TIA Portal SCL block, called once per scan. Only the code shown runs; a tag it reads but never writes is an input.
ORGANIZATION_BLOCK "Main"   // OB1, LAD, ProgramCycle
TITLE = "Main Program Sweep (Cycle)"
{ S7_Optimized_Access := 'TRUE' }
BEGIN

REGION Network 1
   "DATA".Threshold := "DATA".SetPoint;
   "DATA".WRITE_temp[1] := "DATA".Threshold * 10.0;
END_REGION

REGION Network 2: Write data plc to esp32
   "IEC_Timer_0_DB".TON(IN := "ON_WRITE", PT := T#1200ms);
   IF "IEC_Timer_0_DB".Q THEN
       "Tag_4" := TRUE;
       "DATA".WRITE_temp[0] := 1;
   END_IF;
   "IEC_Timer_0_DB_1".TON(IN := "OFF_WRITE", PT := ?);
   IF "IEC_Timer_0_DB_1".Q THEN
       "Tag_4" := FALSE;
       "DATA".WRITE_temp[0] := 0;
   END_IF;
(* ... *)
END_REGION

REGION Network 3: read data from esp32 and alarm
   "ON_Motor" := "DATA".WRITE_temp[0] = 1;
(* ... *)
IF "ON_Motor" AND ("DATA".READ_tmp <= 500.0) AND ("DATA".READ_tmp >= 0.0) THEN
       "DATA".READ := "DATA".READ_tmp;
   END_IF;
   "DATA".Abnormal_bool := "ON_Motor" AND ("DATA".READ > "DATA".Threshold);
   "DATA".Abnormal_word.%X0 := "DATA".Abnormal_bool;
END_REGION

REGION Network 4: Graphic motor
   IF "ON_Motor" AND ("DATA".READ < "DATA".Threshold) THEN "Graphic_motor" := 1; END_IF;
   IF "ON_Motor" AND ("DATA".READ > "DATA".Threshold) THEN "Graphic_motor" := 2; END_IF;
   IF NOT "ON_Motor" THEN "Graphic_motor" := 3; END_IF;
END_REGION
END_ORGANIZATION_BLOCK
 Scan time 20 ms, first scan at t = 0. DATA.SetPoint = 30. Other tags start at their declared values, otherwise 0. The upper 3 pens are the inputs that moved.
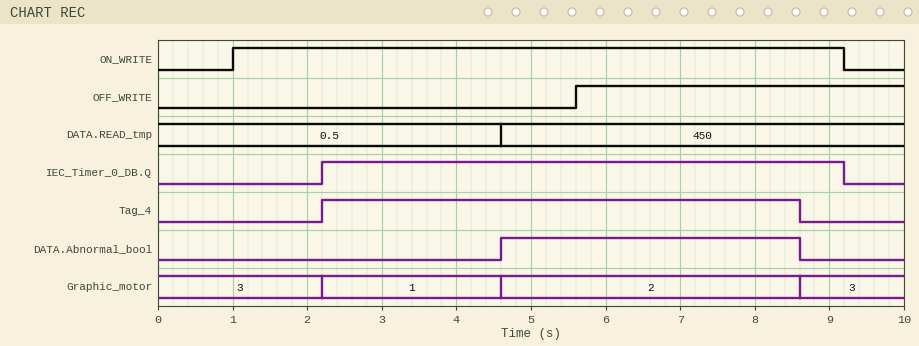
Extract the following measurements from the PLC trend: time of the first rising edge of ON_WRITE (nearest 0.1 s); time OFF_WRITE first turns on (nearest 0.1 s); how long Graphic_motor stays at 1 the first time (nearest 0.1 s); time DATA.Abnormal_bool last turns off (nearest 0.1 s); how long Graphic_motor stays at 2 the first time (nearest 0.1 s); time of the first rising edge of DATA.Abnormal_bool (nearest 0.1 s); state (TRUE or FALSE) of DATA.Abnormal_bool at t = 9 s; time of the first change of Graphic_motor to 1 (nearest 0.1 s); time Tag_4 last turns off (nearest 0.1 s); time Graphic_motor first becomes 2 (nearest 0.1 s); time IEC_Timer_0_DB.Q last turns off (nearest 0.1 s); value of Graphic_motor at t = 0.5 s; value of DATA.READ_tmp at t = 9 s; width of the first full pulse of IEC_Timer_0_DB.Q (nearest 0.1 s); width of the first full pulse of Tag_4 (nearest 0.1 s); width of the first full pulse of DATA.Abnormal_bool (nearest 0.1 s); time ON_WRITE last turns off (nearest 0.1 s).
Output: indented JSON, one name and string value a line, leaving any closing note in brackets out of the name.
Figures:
{
  "time of the first rising edge of ON_WRITE": "1.0 s",
  "time OFF_WRITE first turns on": "5.6 s",
  "how long Graphic_motor stays at 1 the first time": "2.4 s",
  "time DATA.Abnormal_bool last turns off": "8.6 s",
  "how long Graphic_motor stays at 2 the first time": "4.0 s",
  "time of the first rising edge of DATA.Abnormal_bool": "4.6 s",
  "state (TRUE or FALSE) of DATA.Abnormal_bool at t = 9 s": "FALSE",
  "time of the first change of Graphic_motor to 1": "2.2 s",
  "time Tag_4 last turns off": "8.6 s",
  "time Graphic_motor first becomes 2": "4.6 s",
  "time IEC_Timer_0_DB.Q last turns off": "9.2 s",
  "value of Graphic_motor at t = 0.5 s": "3",
  "value of DATA.READ_tmp at t = 9 s": "450",
  "width of the first full pulse of IEC_Timer_0_DB.Q": "7.0 s",
  "width of the first full pulse of Tag_4": "6.4 s",
  "width of the first full pulse of DATA.Abnormal_bool": "4.0 s",
  "time ON_WRITE last turns off": "9.2 s"
}
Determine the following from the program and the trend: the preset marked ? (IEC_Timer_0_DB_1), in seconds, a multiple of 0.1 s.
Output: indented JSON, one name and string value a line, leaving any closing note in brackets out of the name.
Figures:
{
  "the preset marked ? (IEC_Timer_0_DB_1), in seconds, a multiple of 0.1 s": "3.0 s"
}
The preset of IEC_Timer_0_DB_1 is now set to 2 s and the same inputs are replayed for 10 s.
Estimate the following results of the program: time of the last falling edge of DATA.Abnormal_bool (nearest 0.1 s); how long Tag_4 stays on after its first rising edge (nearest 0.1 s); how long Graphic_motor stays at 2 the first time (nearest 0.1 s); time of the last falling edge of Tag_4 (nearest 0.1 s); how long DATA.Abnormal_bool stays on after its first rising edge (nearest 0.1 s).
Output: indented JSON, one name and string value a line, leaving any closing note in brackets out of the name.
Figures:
{
  "time of the last falling edge of DATA.Abnormal_bool": "7.6 s",
  "how long Tag_4 stays on after its first rising edge": "5.4 s",
  "how long Graphic_motor stays at 2 the first time": "3.0 s",
  "time of the last falling edge of Tag_4": "7.6 s",
  "how long DATA.Abnormal_bool stays on after its first rising edge": "3.0 s"
}
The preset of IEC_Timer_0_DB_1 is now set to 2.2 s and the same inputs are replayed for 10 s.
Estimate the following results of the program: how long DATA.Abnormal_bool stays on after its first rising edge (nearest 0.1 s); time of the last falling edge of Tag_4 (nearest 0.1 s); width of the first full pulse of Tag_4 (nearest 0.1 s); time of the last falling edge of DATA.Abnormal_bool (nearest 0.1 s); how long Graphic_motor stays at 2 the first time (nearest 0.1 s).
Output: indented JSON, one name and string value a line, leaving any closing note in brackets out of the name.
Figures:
{
  "how long DATA.Abnormal_bool stays on after its first rising edge": "3.2 s",
  "time of the last falling edge of Tag_4": "7.8 s",
  "width of the first full pulse of Tag_4": "5.6 s",
  "time of the last falling edge of DATA.Abnormal_bool": "7.8 s",
  "how long Graphic_motor stays at 2 the first time": "3.2 s"
}
